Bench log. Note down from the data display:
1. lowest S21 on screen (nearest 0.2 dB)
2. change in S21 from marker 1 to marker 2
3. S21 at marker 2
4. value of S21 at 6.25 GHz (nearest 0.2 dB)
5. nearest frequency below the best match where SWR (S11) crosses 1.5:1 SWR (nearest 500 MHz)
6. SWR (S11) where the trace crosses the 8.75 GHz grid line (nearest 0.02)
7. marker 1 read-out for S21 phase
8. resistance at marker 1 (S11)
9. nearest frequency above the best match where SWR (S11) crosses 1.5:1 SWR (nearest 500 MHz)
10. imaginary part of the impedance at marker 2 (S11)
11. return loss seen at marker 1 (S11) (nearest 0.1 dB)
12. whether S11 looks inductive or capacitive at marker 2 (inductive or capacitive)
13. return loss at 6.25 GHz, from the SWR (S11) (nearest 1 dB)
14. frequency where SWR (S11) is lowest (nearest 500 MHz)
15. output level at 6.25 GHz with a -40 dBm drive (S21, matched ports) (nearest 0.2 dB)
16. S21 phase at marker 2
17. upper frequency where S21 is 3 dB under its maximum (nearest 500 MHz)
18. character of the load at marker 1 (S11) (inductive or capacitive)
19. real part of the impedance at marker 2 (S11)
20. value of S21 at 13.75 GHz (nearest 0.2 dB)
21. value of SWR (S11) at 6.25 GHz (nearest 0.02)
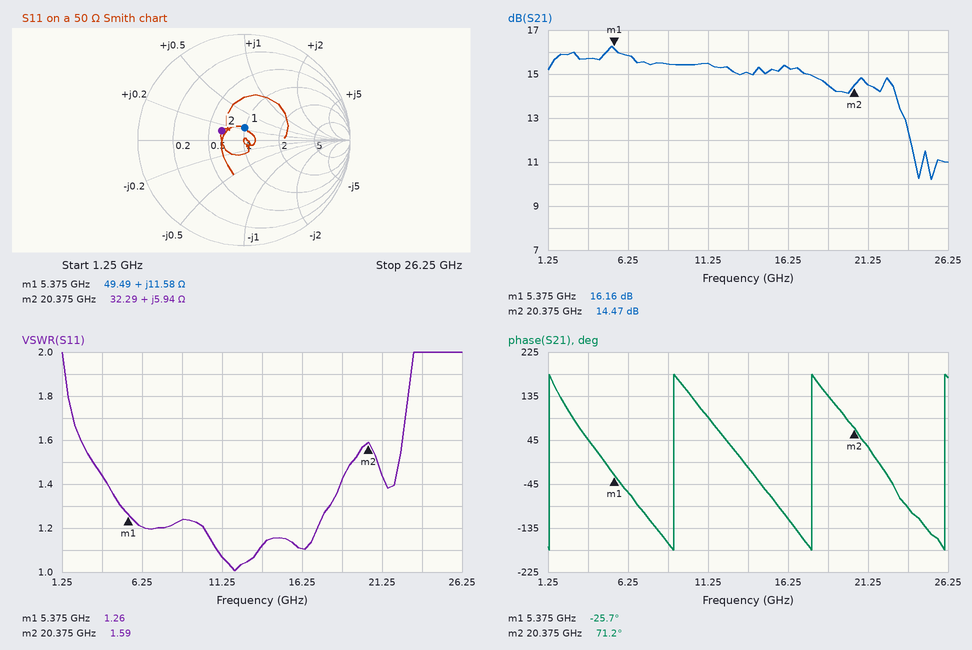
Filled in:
10.2 dB
-1.69 dB
14.47 dB
15.8 dB
3.0 GHz
1.24
-25.7°
49.49 Ω
19.5 GHz
+5.94 Ω
18.7 dB
inductive
21 dB
12.0 GHz
-24.2 dBm
71.2°
23.5 GHz
inductive
32.29 Ω
15.0 dB
1.20
